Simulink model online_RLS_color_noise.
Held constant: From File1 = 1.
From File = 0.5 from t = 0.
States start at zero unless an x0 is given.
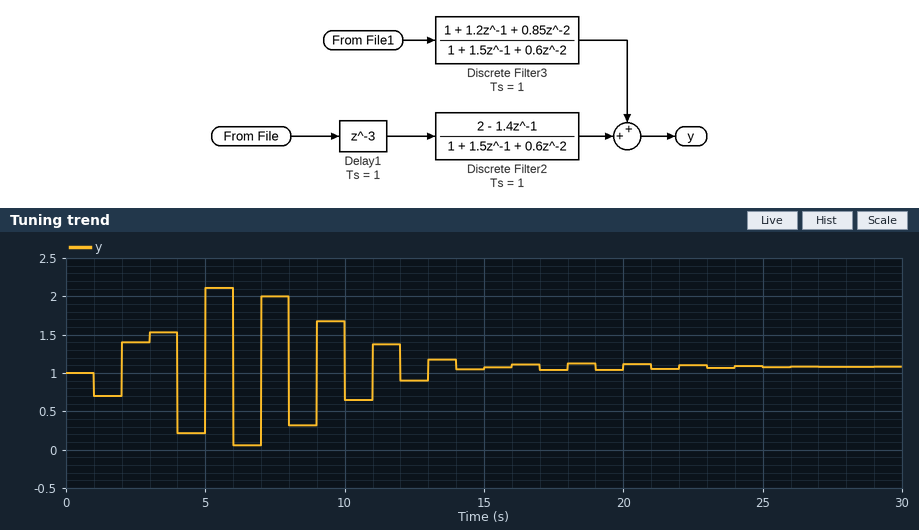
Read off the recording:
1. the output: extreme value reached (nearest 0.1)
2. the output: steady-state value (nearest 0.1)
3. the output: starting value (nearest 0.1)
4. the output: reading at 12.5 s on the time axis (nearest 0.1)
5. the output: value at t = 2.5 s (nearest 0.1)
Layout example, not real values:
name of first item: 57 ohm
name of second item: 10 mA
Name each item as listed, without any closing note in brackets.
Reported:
the output: extreme value reached: 2.1
the output: steady-state value: 1.1
the output: starting value: 1.0
the output: reading at 12.5 s on the time axis: 0.9
the output: value at t = 2.5 s: 1.4
